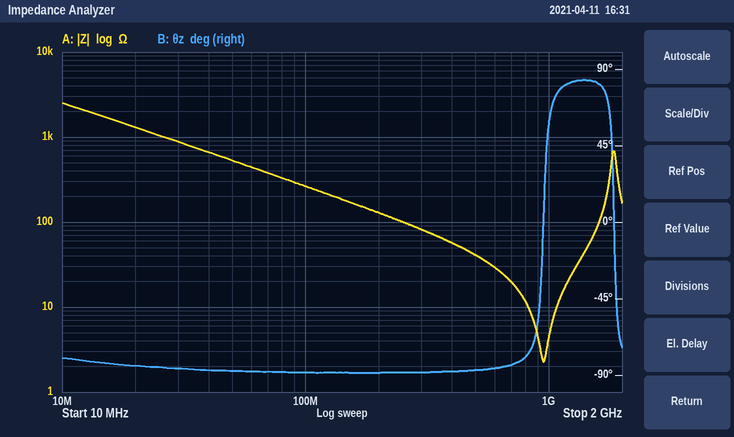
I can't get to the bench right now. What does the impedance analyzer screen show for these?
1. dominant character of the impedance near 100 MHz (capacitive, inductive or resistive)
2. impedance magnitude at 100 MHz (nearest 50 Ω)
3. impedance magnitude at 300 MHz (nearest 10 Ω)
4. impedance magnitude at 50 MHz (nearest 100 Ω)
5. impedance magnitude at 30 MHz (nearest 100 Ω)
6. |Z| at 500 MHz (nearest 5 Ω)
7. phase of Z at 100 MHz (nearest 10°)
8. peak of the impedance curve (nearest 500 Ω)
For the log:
capacitive
250 Ω
80 Ω
500 Ω
900 Ω
40 Ω
-90°
2.5 kΩ
